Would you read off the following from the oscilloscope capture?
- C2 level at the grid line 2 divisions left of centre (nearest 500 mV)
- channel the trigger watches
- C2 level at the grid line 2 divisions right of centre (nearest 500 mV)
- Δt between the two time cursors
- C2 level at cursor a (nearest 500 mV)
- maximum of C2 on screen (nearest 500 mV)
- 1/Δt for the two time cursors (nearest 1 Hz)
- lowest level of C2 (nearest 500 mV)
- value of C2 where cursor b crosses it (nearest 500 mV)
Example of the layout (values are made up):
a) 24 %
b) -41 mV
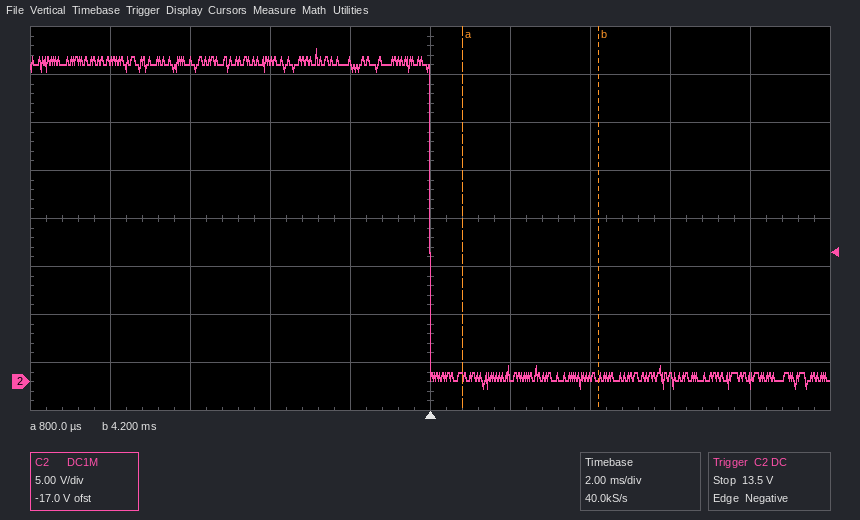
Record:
a) 33.5 V
b) C2
c) 500 mV
d) 3.4 ms
e) 500 mV
f) 34.5 V
g) 294 Hz
h) -500 mV
i) 500 mV
